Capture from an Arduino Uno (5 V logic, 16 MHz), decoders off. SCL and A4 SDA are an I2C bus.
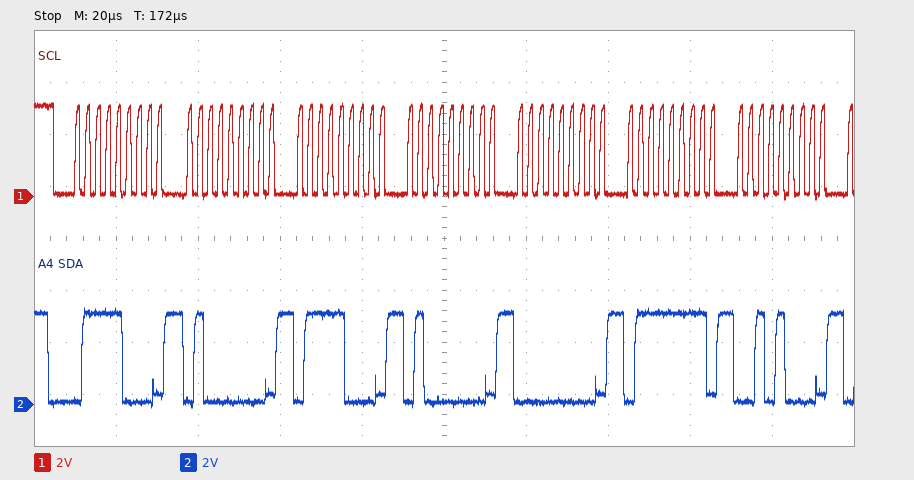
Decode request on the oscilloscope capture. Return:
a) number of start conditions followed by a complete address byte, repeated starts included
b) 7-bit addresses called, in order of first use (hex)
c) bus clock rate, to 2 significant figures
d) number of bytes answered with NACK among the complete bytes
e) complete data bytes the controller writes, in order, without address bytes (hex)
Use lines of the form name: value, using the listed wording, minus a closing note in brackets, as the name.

number of start conditions followed by a complete address byte, repeated starts included: 1
7-bit addresses called, in order of first use: 0x3C
bus clock rate, to 2 significant figures: 400 kHz
number of bytes answered with NACK among the complete bytes: 0
complete data bytes the controller writes, in order, without address bytes: 40 78 40 00 7F 28
